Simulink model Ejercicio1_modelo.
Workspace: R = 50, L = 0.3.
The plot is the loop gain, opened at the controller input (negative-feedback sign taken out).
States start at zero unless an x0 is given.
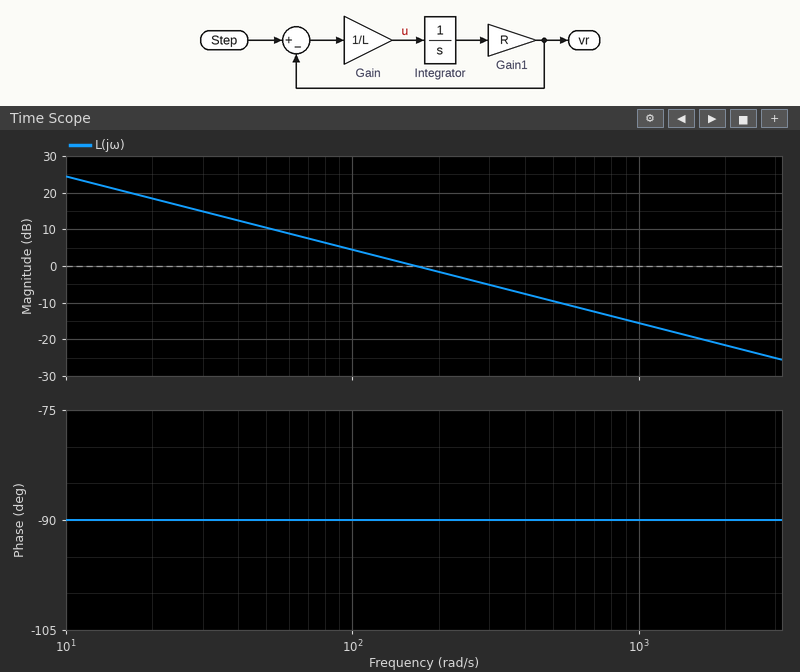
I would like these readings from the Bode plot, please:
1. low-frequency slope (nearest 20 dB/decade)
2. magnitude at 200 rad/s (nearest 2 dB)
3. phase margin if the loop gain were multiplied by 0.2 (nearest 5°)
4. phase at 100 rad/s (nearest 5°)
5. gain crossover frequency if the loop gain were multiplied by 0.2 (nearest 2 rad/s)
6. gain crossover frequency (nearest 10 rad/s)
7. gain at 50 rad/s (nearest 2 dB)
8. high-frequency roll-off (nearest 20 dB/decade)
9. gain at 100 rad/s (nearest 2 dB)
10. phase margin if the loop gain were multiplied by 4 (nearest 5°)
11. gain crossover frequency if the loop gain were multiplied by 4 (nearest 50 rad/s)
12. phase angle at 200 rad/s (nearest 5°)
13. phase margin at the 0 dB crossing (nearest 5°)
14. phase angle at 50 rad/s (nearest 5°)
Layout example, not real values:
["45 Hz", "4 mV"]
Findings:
["-20 dB/decade", "-2 dB", "90°", "-90°", "34 rad/s", "170 rad/s", "10 dB", "-20 dB/decade", "4 dB", "90°", "650 rad/s", "-90°", "90°", "-90°"]
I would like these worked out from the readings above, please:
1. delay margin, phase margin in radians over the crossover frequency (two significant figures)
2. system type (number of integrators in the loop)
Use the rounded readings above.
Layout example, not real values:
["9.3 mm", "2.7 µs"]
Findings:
["0.0092 s", "1"]
